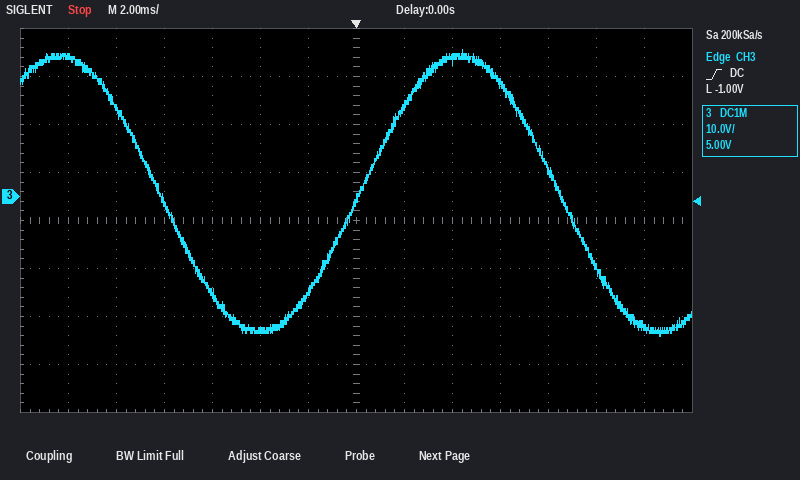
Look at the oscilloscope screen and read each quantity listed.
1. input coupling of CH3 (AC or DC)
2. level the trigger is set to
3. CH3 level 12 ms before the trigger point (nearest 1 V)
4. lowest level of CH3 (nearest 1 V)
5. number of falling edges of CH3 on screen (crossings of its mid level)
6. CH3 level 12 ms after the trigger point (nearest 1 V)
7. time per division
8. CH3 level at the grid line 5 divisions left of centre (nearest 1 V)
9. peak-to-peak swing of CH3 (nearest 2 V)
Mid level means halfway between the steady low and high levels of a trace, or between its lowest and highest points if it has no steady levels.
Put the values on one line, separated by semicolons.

DC; -1.00 V; 29 V; -29 V; 2; -27 V; 2 ms; 18 V; 60 V
